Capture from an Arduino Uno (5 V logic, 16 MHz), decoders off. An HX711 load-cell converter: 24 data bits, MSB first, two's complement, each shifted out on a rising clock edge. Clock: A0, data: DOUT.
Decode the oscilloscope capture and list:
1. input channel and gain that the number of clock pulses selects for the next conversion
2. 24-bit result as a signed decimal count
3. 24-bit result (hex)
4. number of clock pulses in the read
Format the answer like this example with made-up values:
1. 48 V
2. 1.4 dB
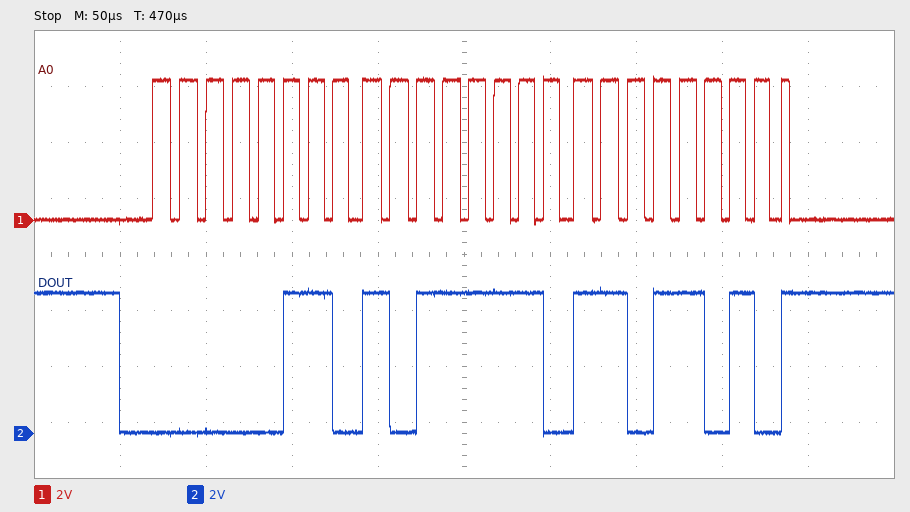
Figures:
1. channel A, gain 128
2. 442074
3. 0x06BEDA
4. 25
